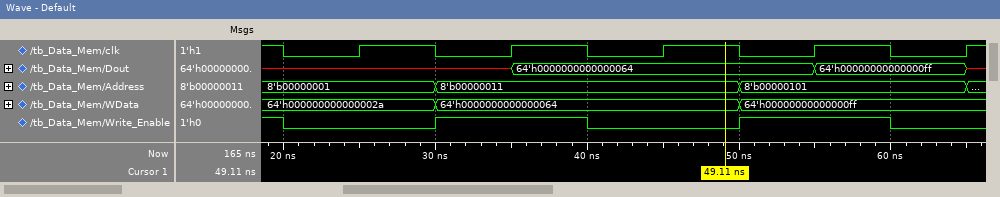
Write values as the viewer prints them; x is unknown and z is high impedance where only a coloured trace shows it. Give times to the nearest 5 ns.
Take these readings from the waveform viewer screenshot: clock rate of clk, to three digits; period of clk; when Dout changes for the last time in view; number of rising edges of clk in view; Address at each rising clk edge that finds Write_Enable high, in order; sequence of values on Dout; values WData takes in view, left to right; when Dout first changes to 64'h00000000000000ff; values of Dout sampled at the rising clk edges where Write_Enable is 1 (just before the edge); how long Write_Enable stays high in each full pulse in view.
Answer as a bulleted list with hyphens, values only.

- 100 MHz
- 10 ns
- 65 ns
- 5
- 8'b00000011, 8'b00000101
- x, 64'h0000000000000064, 64'h00000000000000ff, x
- 64'h000000000000002a, 64'h0000000000000064, 64'h00000000000000ff
- 55 ns
- x, 64'h0000000000000064
- 10 ns, 10 ns
